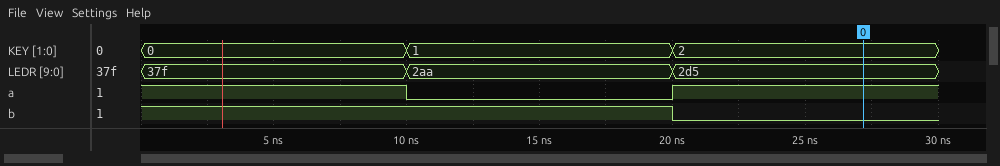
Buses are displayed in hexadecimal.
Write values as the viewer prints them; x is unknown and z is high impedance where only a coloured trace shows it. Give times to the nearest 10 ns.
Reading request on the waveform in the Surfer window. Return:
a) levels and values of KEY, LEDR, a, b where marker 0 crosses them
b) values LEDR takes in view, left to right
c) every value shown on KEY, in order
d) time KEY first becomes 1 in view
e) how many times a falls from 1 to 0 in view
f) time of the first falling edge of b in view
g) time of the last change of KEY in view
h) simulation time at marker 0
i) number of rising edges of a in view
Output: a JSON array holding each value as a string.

["KEY=2, LEDR=2d5, a=1, b=0", "37f, 2aa, 2d5", "0, 1, 2", "10 ns", "1", "20 ns", "20 ns", "30 ns", "1"]
